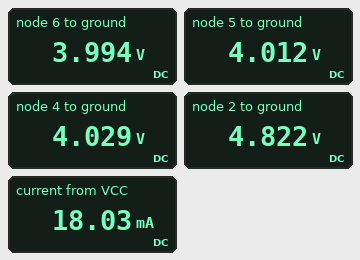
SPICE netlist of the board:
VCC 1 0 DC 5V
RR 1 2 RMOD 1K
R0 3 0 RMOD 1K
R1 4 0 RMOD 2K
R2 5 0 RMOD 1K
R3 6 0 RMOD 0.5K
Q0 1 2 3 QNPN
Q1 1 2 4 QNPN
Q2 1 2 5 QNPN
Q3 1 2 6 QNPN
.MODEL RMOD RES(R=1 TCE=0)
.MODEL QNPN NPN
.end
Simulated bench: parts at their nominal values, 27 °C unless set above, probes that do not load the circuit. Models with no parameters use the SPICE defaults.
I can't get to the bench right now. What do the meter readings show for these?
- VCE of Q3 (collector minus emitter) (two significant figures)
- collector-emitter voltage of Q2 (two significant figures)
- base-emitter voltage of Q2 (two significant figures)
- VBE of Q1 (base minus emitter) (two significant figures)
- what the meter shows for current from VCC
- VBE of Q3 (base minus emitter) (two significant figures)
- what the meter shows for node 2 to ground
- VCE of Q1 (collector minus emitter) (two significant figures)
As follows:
1.0 V
990 mV
810 mV
790 mV
18.03 mA
830 mV
4.822 V
970 mV
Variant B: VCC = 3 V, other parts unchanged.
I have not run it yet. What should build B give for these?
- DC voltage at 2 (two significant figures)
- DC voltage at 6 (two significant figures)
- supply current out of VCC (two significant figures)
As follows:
2.9 V
2.1 V
9.5 mA
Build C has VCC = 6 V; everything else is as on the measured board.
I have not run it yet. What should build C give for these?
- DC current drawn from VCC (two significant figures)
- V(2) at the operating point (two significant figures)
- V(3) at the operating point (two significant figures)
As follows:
22 mA
5.8 V
5.0 V
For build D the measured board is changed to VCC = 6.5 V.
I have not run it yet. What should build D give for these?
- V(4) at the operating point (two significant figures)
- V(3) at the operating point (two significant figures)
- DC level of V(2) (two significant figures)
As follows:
5.5 V
5.4 V
6.3 V
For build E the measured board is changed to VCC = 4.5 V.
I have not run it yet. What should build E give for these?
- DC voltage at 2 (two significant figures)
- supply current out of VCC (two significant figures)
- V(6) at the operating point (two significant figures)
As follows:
4.3 V
16 mA
3.5 V
